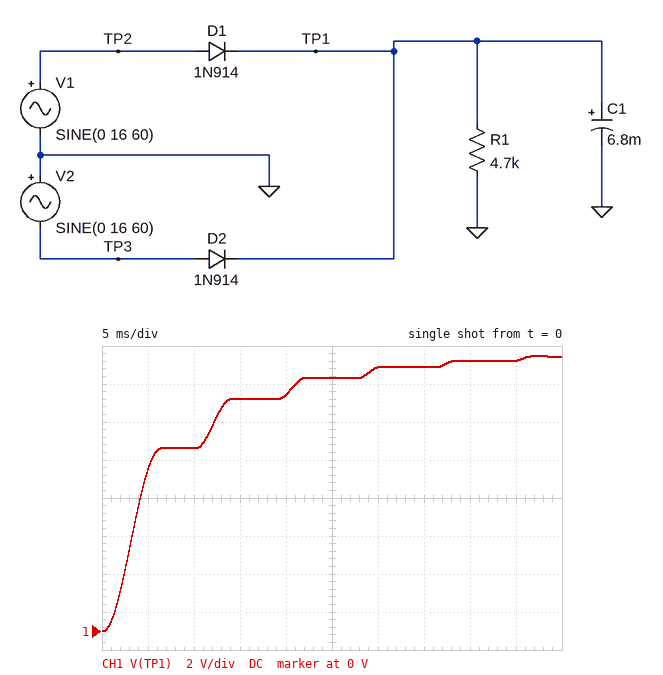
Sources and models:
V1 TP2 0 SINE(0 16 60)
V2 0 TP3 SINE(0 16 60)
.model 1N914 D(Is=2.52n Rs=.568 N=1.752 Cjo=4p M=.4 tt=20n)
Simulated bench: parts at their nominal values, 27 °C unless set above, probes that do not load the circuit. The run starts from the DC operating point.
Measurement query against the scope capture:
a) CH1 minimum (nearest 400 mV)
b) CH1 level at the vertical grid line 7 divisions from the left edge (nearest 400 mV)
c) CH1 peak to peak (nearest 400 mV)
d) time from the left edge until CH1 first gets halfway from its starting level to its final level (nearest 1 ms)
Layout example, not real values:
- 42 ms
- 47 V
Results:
- 0 V
- 14.0 V
- 14.4 V
- 4 ms
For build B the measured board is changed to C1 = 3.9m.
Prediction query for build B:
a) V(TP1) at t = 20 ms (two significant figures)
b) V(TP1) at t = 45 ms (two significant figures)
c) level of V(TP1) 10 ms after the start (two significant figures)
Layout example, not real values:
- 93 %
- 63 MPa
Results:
- 14 V
- 15 V
- 12 V
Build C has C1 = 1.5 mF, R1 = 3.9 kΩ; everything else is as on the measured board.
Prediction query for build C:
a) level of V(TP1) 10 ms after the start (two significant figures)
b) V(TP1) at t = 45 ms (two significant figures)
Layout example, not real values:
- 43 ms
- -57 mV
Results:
- 14 V
- 15 V
